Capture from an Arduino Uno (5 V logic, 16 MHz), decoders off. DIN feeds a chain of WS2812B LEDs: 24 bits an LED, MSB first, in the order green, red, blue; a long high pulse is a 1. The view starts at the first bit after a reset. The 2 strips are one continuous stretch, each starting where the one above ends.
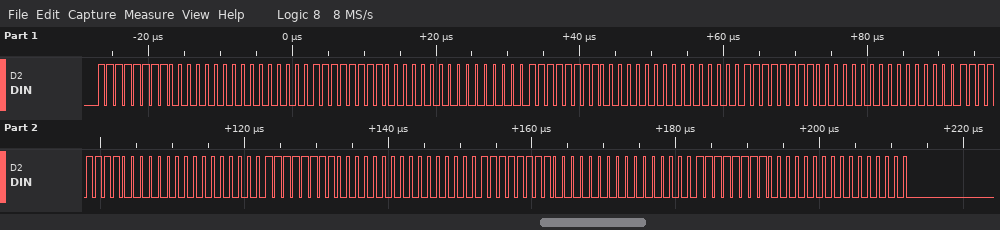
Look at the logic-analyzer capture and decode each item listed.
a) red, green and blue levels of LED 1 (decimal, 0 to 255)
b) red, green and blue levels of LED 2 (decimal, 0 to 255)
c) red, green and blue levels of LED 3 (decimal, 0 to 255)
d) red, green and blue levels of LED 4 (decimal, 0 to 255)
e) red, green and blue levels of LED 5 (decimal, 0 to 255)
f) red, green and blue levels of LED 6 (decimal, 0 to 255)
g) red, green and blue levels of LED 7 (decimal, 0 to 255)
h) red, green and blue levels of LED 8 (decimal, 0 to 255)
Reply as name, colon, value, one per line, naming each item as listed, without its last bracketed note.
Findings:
red, green and blue levels of LED 1: 0, 255, 0
red, green and blue levels of LED 2: 0, 255, 0
red, green and blue levels of LED 3: 0, 255, 0
red, green and blue levels of LED 4: 0, 255, 0
red, green and blue levels of LED 5: 0, 255, 0
red, green and blue levels of LED 6: 0, 255, 0
red, green and blue levels of LED 7: 0, 255, 0
red, green and blue levels of LED 8: 0, 255, 0
